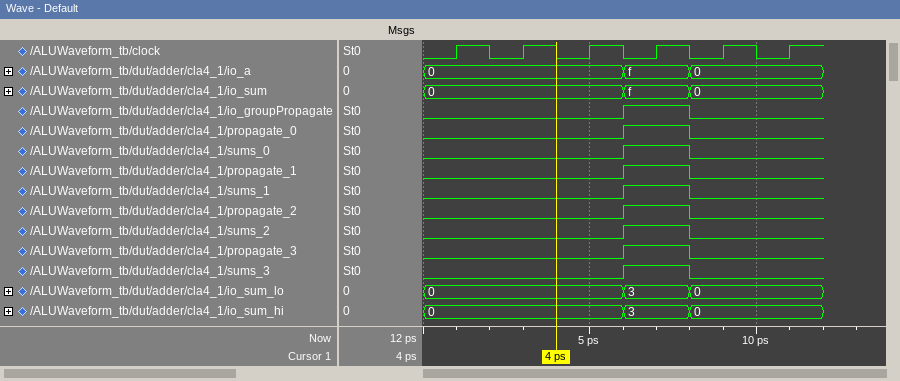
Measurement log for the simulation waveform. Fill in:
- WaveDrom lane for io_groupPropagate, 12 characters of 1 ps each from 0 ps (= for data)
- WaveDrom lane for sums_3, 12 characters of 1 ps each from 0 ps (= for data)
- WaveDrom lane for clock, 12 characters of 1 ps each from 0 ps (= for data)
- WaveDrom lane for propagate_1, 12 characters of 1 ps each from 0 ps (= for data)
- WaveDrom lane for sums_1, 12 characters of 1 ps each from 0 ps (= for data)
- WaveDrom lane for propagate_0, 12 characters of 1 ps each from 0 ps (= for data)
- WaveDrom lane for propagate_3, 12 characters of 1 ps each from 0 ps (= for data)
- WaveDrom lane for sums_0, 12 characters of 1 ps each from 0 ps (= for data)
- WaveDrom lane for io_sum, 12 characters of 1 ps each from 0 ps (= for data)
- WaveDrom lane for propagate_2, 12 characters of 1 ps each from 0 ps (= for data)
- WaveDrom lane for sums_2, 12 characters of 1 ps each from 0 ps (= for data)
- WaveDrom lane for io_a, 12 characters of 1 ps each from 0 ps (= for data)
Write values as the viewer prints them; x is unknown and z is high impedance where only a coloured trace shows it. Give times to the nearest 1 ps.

{name: 'io_groupPropagate', wave: '0.....1.0...'}
{name: 'sums_3', wave: '0.....1.0...'}
{name: 'clock', wave: '010101010101'}
{name: 'propagate_1', wave: '0.....1.0...'}
{name: 'sums_1', wave: '0.....1.0...'}
{name: 'propagate_0', wave: '0.....1.0...'}
{name: 'propagate_3', wave: '0.....1.0...'}
{name: 'sums_0', wave: '0.....1.0...'}
{name: 'io_sum', wave: '=.....=.=...', data: '0 f 0'}
{name: 'propagate_2', wave: '0.....1.0...'}
{name: 'sums_2', wave: '0.....1.0...'}
{name: 'io_a', wave: '=.....=.=...', data: '0 f 0'}
